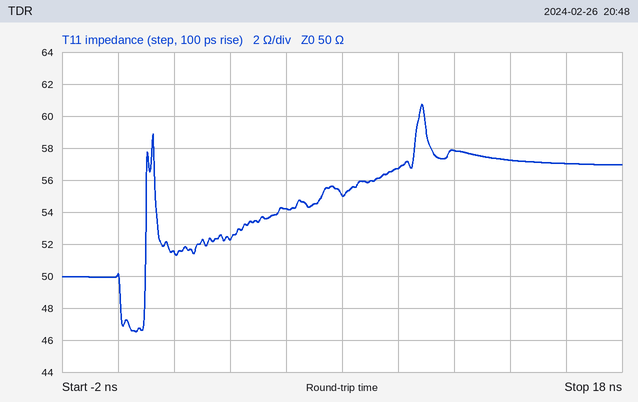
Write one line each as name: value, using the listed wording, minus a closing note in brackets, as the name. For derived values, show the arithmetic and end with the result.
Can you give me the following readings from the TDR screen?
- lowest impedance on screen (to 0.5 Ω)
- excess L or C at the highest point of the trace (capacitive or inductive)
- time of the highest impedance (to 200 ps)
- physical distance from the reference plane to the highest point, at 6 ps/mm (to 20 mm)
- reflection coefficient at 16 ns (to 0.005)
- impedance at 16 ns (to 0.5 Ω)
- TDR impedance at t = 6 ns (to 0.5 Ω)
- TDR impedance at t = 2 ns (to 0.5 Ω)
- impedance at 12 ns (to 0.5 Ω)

lowest impedance on screen: 46.5 Ω
excess L or C at the highest point of the trace: inductive
time of the highest impedance: 10.8 ns
physical distance from the reference plane to the highest point, at 6 ps/mm: 10.8 ns / 2 / 6 ps/mm ≈ 900 mm
reflection coefficient at 16 ns: (57 − 50)/(57 + 50) ≈ +0.065
impedance at 16 ns: 57.0 Ω
TDR impedance at t = 6 ns: 54.0 Ω
TDR impedance at t = 2 ns: 51.5 Ω
impedance at 12 ns: 58.0 Ω
